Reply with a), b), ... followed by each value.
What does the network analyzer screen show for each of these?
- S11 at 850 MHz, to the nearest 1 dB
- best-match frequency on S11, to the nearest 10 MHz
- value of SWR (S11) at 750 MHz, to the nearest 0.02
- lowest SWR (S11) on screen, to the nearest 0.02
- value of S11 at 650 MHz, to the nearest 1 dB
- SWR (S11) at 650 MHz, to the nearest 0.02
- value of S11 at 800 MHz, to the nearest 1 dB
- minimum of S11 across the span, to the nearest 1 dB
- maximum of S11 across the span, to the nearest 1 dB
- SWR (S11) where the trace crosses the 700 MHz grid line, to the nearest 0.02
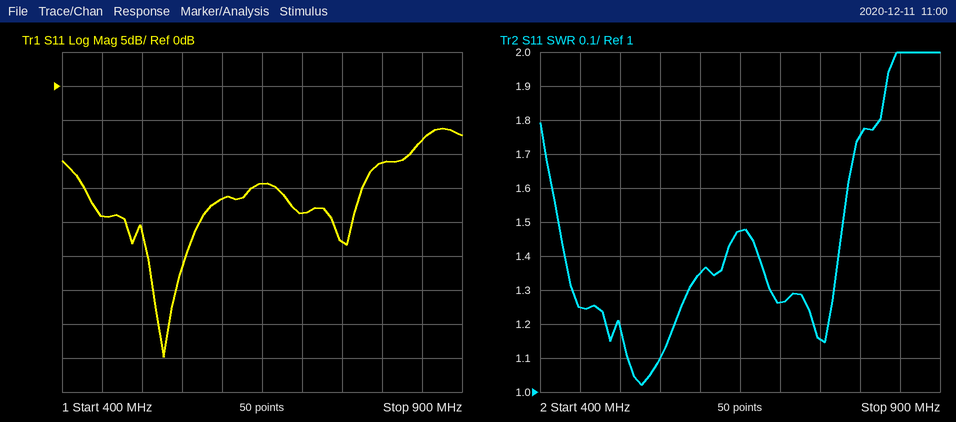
a) -8 dB
b) 530 MHz
c) 1.16
d) 1.02
e) -14 dB
f) 1.48
g) -11 dB
h) -40 dB
i) -6 dB
j) 1.26
